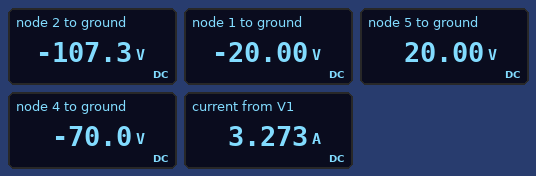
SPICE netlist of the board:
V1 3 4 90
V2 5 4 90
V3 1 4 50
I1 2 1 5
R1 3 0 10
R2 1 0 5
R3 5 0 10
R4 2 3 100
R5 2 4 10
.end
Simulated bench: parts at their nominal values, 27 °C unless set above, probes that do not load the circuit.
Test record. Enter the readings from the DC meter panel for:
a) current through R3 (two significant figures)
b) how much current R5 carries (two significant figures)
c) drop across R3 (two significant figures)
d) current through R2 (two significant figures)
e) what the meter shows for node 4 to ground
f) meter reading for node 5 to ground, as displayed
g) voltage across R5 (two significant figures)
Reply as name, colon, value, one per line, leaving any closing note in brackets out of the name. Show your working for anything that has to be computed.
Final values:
current through R3: (20 V) / 10 Ω = 2.0 A
how much current R5 carries: (-70 V - (-107.3 V)) / 10 Ω = 3.7 A
drop across R3: 20 V = 20 V
current through R2: (0 V - (-20 V)) / 5 Ω = 4.0 A
what the meter shows for node 4 to ground: -70.0 V
meter reading for node 5 to ground, as displayed: 20.00 V
voltage across R5: -70 V - (-107.3 V) = 37 V
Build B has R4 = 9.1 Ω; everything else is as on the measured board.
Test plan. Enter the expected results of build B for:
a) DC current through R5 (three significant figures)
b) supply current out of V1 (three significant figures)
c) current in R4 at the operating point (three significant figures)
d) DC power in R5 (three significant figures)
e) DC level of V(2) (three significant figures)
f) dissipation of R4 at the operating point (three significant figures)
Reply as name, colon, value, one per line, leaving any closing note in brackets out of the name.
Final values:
DC current through R5: 2.33 A
supply current out of V1: 9.33 A
current in R4 at the operating point: 7.33 A
DC power in R5: 54.3 W
DC level of V(2): -46.7 V
dissipation of R4 at the operating point: 489 W
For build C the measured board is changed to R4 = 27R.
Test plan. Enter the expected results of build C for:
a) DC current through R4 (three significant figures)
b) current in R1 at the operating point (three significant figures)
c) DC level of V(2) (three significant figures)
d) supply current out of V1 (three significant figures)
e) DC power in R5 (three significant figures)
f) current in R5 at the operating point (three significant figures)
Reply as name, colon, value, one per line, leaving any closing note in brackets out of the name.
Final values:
DC current through R4: 3.78 A
current in R1 at the operating point: 2.00 A
DC level of V(2): -82.2 V
supply current out of V1: 5.78 A
DC power in R5: 14.8 W
current in R5 at the operating point: 1.22 A
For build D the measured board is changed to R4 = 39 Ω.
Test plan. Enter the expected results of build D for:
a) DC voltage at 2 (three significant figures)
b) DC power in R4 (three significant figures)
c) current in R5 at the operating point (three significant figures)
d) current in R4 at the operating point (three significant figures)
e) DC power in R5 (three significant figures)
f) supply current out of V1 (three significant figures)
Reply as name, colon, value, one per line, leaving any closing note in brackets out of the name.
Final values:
DC voltage at 2: -91.4 V
DC power in R4: 318 W
current in R5 at the operating point: 2.14 A
current in R4 at the operating point: 2.86 A
DC power in R5: 45.9 W
supply current out of V1: 4.86 A
